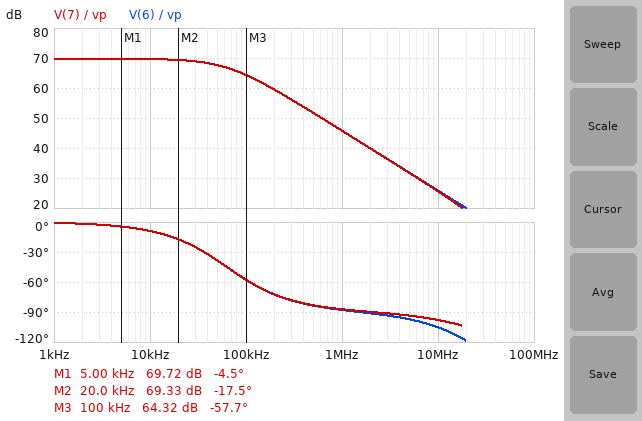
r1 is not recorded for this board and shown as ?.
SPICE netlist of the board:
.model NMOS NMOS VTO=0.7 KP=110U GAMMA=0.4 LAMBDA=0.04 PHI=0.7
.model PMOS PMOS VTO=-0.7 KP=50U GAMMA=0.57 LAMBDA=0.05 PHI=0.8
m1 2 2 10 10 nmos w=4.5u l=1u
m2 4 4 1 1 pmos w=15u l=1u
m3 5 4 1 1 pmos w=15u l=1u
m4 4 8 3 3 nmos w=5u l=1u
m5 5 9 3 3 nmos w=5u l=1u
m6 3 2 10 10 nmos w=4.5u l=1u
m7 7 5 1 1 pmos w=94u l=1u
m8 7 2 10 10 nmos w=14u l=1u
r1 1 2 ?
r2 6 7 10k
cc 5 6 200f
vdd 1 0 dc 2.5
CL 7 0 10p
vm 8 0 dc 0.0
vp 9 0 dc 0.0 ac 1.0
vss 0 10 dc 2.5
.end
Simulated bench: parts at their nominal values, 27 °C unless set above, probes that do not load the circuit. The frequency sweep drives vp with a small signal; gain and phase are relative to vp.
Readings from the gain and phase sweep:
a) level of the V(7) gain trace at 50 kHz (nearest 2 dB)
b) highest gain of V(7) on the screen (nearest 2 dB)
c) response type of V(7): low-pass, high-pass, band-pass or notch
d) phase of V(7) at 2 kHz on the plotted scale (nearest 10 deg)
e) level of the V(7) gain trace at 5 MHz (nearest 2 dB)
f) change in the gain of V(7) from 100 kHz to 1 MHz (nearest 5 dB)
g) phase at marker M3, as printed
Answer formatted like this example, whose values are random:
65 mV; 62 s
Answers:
68 dB; 70 dB; low-pass; 0 deg; 32 dB; -20 dB; -57.7 deg
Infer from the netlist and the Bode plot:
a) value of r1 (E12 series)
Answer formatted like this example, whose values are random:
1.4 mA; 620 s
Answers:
27 kΩ
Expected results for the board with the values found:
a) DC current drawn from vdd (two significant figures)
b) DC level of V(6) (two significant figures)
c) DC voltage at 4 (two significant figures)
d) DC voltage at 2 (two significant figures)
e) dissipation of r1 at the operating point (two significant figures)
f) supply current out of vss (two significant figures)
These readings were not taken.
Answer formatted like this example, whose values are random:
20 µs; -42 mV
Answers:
700 µA; 340 mV; 1.4 V; -1.1 V; 480 µW; 700 µA
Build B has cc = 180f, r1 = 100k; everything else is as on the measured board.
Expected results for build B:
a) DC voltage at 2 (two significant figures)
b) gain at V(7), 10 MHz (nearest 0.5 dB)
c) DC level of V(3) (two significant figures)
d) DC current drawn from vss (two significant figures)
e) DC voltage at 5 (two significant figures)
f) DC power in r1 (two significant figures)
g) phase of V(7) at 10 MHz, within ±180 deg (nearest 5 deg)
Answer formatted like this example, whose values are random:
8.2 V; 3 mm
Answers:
-1.4 V; 21.0 dB; -960 mV; 210 µA; 1.6 V; 150 µW; -110 deg
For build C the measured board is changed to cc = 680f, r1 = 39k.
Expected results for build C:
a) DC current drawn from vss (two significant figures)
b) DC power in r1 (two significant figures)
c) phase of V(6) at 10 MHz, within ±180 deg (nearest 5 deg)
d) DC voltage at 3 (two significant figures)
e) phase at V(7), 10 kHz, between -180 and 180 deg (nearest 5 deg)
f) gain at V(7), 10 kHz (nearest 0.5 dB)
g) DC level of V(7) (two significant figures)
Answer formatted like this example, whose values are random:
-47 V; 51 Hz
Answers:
500 µA; 350 µW; -110 deg; -1.1 V; -40 deg; 70.5 dB; 410 mV
